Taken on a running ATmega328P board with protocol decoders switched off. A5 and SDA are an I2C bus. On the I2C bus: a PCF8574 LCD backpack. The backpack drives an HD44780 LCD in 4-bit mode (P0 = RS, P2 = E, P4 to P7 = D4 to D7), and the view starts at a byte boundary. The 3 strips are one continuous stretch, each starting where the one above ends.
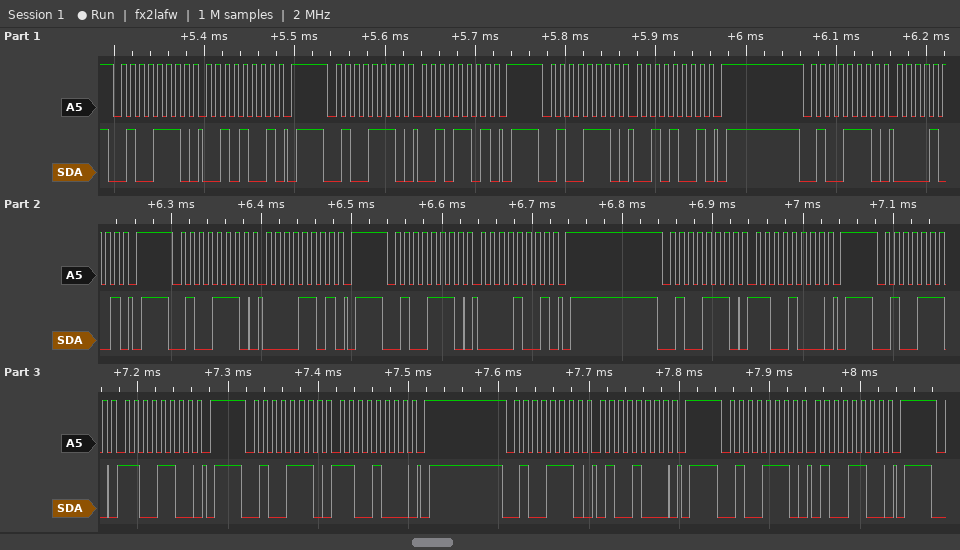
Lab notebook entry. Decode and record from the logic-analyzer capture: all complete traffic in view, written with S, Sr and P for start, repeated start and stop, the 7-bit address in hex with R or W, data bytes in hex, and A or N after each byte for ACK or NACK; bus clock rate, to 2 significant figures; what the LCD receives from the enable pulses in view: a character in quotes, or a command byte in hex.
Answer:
S 27W A 29 A P S 27W A 2D A P S 27W A 29 A P S 27W A 09 A P S 27W A 0D A P S 27W A 09 A P S 27W A C8 A P S 27W A CC A P S 27W A C8 A P S 27W A 48 A P S 27W A 4C A P
100 kHz
' '
